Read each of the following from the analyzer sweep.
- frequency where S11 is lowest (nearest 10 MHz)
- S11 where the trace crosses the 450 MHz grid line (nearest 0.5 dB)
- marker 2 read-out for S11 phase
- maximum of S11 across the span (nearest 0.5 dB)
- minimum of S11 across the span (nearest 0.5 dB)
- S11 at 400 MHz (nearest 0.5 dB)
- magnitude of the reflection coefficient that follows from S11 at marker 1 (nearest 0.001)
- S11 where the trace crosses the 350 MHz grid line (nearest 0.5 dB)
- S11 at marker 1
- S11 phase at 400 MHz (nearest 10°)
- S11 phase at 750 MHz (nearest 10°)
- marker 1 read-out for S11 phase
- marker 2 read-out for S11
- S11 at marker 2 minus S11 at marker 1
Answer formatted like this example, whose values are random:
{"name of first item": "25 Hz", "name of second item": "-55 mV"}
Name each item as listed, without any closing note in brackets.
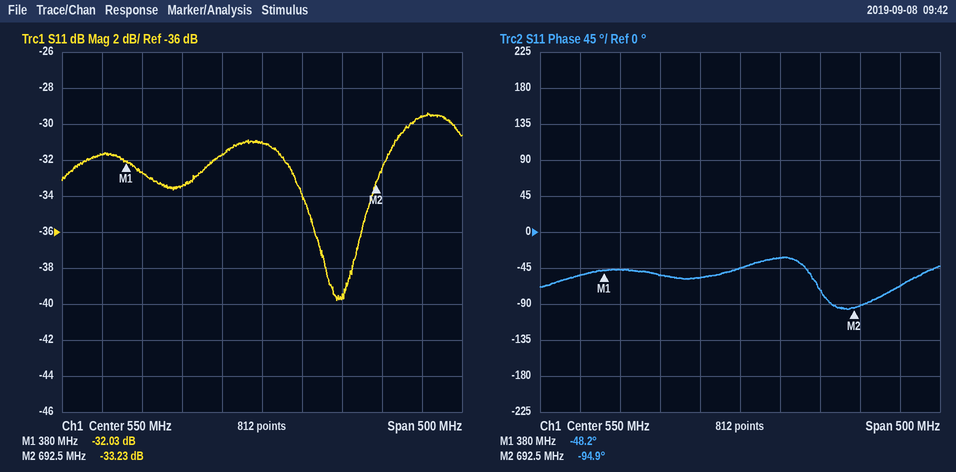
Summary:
{"frequency where S11 is lowest": "640 MHz", "S11 where the trace crosses the 450 MHz grid line": "-33.5 dB", "marker 2 read-out for S11 phase": "-94.9°", "maximum of S11 across the span": "-29.5 dB", "minimum of S11 across the span": "-40.0 dB", "S11 at 400 MHz": "-32.5 dB", "magnitude of the reflection coefficient that follows from S11 at marker 1": "0.025", "S11 where the trace crosses the 350 MHz grid line": "-31.5 dB", "S11 at marker 1": "-32.03 dB", "S11 phase at 400 MHz": "-50°", "S11 phase at 750 MHz": "-70°", "marker 1 read-out for S11 phase": "-48.2°", "marker 2 read-out for S11": "-33.23 dB", "S11 at marker 2 minus S11 at marker 1": "-1.20 dB"}
